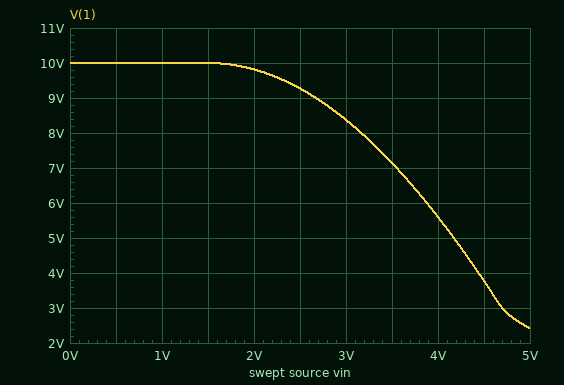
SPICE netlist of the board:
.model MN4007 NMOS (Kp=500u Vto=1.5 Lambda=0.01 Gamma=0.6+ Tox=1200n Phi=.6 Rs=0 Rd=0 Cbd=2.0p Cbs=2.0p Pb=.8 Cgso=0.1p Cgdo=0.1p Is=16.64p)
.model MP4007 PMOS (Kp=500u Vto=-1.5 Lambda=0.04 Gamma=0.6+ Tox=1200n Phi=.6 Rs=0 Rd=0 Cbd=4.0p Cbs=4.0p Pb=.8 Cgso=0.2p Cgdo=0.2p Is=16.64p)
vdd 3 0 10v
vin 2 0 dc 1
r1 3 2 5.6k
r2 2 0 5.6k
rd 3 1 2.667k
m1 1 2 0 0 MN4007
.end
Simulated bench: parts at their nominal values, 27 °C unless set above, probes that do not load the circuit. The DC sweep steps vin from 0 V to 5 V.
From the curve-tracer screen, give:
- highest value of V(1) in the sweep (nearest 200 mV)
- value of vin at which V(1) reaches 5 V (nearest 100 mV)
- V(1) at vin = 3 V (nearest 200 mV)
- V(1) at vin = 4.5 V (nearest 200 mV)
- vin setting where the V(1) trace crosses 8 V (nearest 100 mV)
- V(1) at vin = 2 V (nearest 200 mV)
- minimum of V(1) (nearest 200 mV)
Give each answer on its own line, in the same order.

10.0 V
4.2 V
8.4 V
3.8 V
3.2 V
9.8 V
2.4 V
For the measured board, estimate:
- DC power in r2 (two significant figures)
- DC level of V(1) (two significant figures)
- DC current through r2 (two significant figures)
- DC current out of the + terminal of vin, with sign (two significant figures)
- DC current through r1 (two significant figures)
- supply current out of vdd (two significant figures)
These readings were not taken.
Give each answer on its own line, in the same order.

180 µW
10 V
180 µA
-1.4 mA
1.6 mA
1.6 mA
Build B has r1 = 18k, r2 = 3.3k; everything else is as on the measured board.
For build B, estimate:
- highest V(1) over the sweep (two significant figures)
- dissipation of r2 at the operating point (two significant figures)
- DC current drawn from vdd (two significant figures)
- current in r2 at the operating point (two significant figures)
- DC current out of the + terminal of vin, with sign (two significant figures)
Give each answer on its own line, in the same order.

10 V
300 µW
500 µA
300 µA
-200 µA
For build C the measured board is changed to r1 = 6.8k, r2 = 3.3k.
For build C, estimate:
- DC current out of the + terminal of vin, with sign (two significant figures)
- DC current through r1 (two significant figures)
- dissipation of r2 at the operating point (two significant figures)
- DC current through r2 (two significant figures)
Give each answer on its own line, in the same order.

-1.0 mA
1.3 mA
300 µW
300 µA
